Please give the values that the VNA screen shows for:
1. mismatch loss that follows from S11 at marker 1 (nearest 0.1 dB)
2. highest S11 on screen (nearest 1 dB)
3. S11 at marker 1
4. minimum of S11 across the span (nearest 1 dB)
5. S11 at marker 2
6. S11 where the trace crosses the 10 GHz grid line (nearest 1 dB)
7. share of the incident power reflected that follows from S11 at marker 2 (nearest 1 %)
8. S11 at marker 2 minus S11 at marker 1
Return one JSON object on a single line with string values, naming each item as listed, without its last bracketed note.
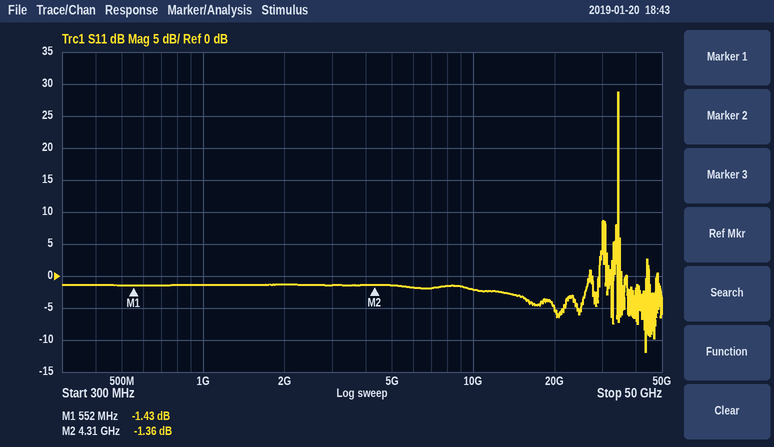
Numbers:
{"mismatch loss that follows from S11 at marker 1": "5.5 dB", "highest S11 on screen": "29 dB", "S11 at marker 1": "-1.43 dB", "minimum of S11 across the span": "-12 dB", "S11 at marker 2": "-1.36 dB", "S11 where the trace crosses the 10 GHz grid line": "-2 dB", "share of the incident power reflected that follows from S11 at marker 2": "73 %", "S11 at marker 2 minus S11 at marker 1": "0.07 dB"}
